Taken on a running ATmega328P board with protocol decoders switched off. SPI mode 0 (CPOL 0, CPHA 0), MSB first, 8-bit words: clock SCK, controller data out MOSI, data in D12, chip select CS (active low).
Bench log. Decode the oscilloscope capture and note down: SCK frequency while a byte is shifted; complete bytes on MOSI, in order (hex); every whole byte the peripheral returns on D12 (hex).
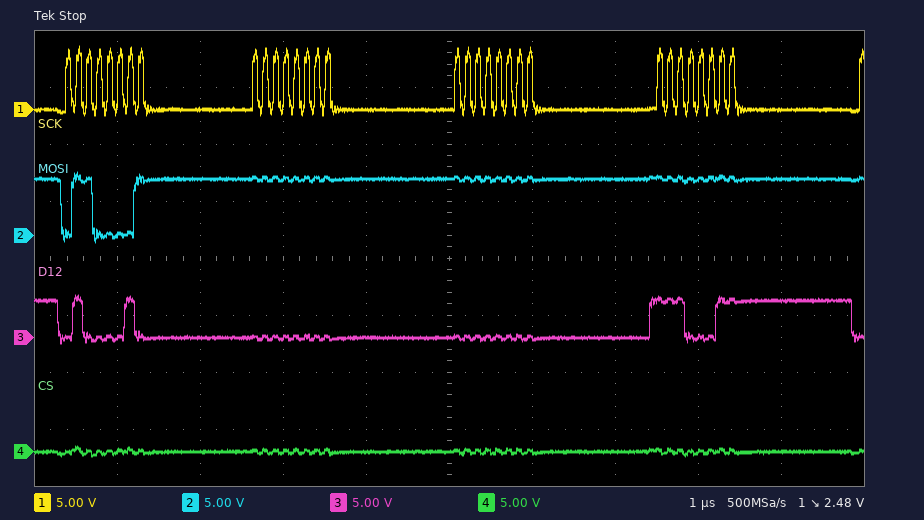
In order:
8 MHz
61 FF FF FF
42 00 00 E3
